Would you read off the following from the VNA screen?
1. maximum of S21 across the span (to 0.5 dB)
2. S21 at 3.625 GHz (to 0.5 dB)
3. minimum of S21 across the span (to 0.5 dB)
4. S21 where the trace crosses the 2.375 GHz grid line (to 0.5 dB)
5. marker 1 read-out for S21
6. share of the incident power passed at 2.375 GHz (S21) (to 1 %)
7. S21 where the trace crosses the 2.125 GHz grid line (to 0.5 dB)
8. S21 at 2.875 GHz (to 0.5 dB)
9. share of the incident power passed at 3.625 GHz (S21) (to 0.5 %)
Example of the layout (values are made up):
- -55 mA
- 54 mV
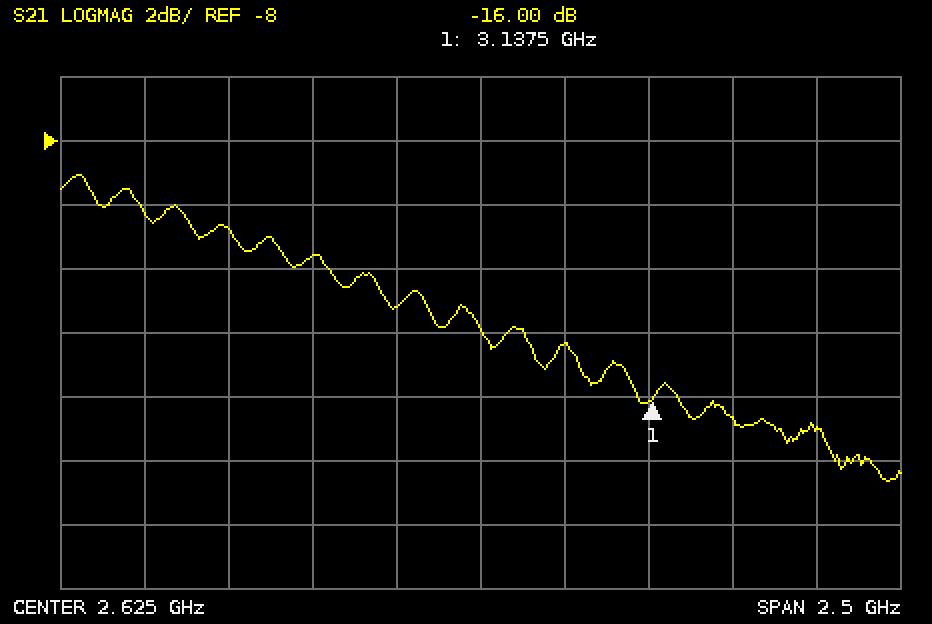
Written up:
- -9.0 dB
- -17.0 dB
- -18.5 dB
- -13.0 dB
- -16.00 dB
- 5 %
- -11.5 dB
- -14.5 dB
- 2.0 %
